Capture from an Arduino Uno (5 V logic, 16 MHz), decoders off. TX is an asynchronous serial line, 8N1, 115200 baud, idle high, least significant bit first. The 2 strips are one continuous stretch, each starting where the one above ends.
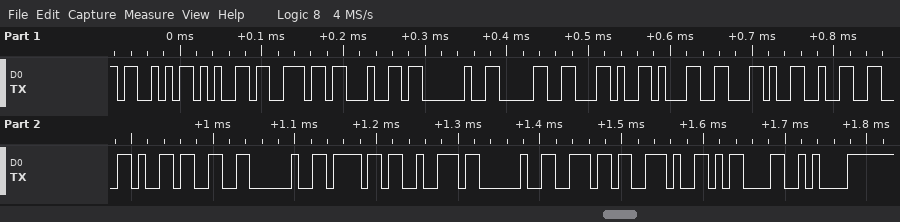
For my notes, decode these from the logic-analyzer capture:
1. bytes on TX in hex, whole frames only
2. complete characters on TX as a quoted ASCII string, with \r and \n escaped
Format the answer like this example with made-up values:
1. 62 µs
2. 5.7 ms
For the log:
1. 53 65 6E 64 20 30 2C 31 2C 32 2C 33 20 6F 72 20 6E 2E 0D 0A
2. "Send 0,1,2,3 or n.\r\n"
